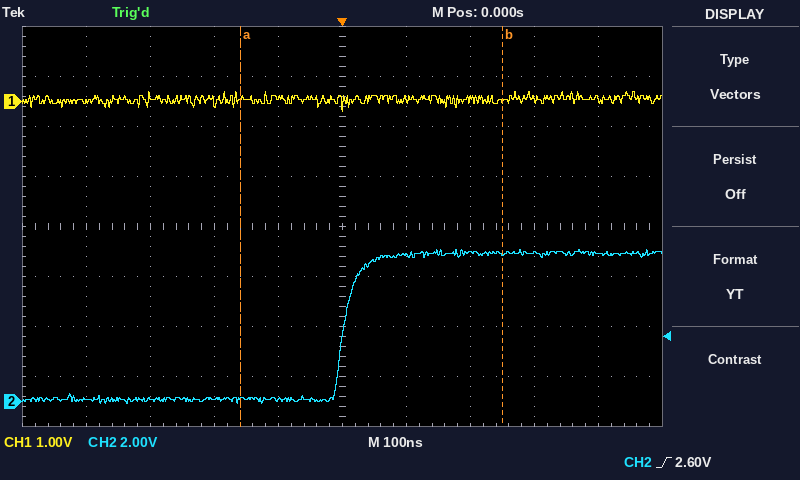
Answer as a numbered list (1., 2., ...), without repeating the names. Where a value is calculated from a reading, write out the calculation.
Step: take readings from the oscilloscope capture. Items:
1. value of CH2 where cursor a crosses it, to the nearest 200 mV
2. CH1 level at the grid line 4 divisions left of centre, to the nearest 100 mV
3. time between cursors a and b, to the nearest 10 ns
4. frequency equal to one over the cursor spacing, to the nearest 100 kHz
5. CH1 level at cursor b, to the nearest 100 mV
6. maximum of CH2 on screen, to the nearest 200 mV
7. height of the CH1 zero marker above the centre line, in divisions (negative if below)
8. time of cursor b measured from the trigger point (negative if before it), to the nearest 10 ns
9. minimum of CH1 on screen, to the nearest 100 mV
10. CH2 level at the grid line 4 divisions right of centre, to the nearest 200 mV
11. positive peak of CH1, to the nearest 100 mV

1. 0.0 V
2. 0.0 V
3. 410 ns
4. 1 / 410 ns ≈ 2.4 MHz
5. 0.0 V
6. 6.0 V
7. +2.5 div
8. +250 ns
9. -200 mV
10. 6.0 V
11. 200 mV
